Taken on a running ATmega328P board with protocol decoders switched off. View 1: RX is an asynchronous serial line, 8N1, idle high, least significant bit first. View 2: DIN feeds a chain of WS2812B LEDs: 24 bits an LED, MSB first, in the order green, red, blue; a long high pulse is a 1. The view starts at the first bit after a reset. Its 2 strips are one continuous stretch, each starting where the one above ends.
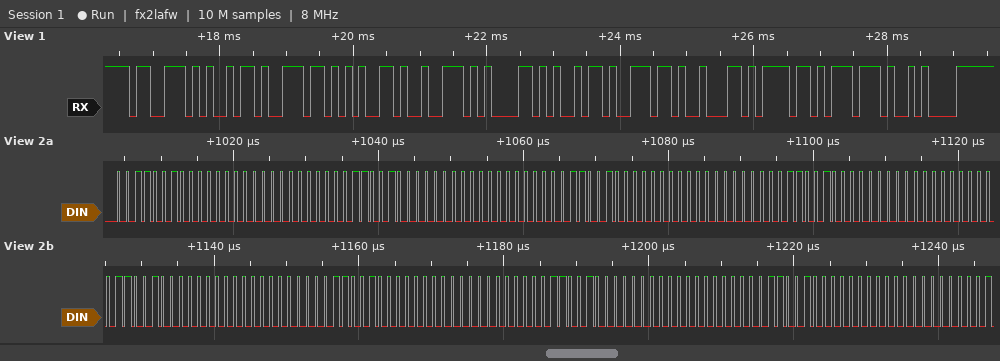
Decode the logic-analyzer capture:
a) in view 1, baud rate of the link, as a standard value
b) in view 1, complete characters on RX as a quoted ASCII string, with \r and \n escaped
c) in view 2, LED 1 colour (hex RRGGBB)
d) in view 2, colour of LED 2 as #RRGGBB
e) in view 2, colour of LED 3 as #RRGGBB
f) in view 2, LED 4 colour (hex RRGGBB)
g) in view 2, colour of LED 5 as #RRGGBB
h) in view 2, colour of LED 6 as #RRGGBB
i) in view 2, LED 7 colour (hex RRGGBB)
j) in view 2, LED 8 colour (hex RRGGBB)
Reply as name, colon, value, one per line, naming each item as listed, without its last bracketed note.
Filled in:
in view 1, baud rate of the link, as a standard value: 9600 baud
in view 1, complete characters on RX as a quoted ASCII string, with \r and \n escaped: "sinerainbow\n"
in view 2, LED 1 colour: #003200
in view 2, colour of LED 2 as #RRGGBB: #003200
in view 2, colour of LED 3 as #RRGGBB: #003200
in view 2, LED 4 colour: #003200
in view 2, colour of LED 5 as #RRGGBB: #003200
in view 2, colour of LED 6 as #RRGGBB: #003200
in view 2, LED 7 colour: #003200
in view 2, LED 8 colour: #003200
